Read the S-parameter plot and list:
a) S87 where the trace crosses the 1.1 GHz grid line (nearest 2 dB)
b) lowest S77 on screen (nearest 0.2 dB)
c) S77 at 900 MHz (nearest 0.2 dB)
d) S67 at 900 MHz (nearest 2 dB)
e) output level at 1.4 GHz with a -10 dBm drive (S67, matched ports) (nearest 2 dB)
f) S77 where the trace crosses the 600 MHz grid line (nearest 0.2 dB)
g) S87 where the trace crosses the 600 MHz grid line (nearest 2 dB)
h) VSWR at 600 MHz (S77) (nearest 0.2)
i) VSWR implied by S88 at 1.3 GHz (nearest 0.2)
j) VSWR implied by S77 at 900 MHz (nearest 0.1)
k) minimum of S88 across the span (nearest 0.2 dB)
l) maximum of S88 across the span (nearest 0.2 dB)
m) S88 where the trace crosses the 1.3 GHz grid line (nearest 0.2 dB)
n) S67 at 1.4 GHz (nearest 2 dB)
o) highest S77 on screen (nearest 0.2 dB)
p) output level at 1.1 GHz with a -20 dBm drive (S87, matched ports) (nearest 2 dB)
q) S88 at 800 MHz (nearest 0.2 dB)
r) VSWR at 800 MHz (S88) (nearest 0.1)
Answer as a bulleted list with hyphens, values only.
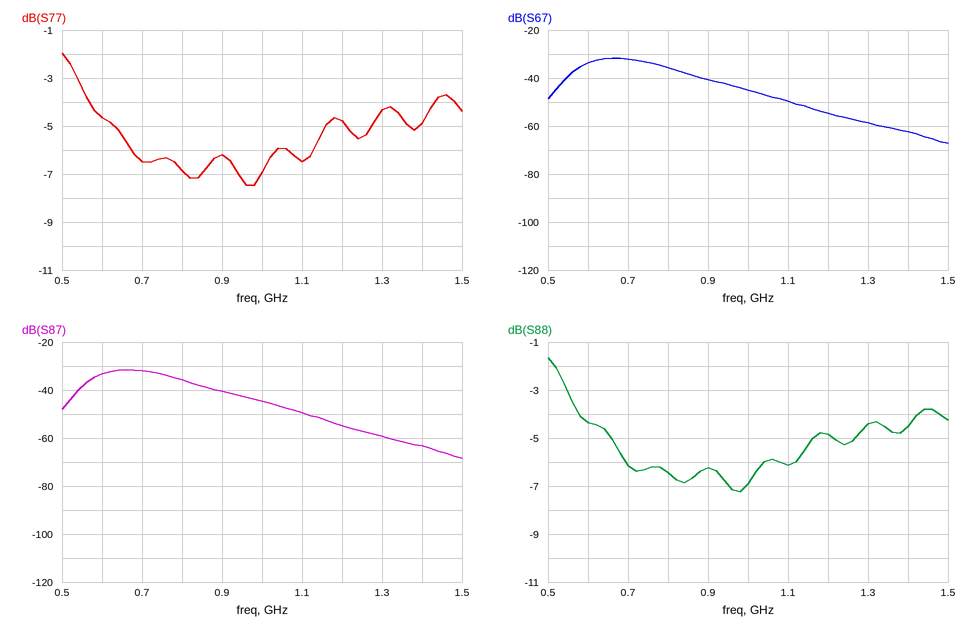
- -50 dB
- -7.4 dB
- -6.2 dB
- -40 dB
- -72 dBm
- -4.6 dB
- -34 dB
- 3.8
- 4.0
- 2.9
- -7.2 dB
- -1.6 dB
- -4.4 dB
- -62 dB
- -2.0 dB
- -70 dBm
- -6.4 dB
- 2.8
